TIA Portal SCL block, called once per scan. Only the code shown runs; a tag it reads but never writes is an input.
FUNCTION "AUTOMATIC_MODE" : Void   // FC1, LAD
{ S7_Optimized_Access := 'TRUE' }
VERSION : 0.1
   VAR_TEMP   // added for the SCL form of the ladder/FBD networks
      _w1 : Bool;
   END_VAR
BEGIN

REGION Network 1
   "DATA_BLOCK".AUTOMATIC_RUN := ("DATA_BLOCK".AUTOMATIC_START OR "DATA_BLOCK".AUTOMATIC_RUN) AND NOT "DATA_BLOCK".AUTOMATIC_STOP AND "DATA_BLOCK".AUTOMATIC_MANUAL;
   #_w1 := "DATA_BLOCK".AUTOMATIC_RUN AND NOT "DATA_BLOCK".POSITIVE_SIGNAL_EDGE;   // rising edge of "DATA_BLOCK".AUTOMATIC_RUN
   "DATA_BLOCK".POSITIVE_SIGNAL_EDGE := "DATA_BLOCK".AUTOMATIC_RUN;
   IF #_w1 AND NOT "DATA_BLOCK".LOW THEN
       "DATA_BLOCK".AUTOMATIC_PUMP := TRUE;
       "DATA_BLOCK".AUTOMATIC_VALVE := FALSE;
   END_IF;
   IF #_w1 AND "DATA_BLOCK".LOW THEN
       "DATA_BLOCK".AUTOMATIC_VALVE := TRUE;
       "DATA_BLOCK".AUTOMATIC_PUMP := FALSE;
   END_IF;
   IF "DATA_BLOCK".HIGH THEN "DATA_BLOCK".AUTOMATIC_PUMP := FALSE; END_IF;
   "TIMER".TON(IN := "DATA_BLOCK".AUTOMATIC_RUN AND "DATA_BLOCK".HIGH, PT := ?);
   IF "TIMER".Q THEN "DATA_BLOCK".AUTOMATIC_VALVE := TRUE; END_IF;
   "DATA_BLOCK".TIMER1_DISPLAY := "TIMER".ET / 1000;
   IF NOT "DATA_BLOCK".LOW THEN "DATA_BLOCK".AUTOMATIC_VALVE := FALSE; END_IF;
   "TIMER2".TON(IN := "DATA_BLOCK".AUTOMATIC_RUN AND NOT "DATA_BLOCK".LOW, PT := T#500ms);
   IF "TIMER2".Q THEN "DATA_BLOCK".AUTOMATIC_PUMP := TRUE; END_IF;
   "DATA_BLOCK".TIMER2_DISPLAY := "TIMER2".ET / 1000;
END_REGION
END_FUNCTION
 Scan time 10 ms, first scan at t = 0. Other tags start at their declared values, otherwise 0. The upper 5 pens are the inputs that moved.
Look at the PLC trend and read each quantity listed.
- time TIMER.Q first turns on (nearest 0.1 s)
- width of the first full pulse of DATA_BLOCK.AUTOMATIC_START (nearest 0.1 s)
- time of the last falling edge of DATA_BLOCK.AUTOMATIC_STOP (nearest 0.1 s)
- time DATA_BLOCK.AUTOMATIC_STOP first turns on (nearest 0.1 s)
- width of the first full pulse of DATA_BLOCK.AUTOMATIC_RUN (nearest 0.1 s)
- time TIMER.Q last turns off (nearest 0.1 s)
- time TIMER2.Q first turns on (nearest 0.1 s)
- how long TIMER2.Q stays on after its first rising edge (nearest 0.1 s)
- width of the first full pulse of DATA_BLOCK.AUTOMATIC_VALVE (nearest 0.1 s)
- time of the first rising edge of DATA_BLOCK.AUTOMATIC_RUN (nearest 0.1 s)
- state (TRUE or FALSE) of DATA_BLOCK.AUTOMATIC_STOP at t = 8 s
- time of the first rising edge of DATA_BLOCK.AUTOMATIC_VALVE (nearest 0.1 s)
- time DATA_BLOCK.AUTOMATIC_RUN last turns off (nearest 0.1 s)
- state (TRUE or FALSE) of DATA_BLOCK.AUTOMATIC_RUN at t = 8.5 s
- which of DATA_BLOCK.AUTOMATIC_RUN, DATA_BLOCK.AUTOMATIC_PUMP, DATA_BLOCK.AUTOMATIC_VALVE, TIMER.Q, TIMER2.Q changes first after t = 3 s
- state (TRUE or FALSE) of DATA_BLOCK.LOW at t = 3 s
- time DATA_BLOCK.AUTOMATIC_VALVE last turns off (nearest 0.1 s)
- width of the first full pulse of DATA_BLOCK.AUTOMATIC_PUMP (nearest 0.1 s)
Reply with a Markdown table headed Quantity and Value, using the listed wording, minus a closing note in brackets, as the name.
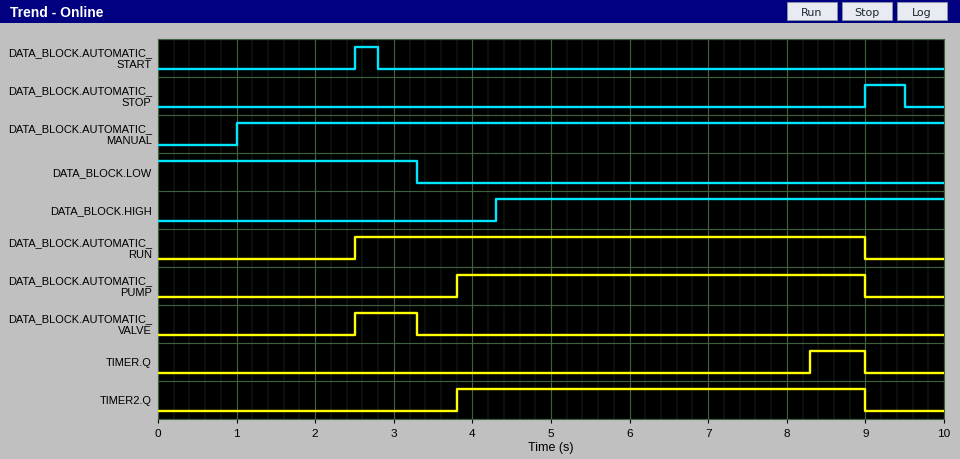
| Quantity | Value |
|---|---|
| time TIMER.Q first turns on | 8.3 s |
| width of the first full pulse of DATA_BLOCK.AUTOMATIC_START | 0.3 s |
| time of the last falling edge of DATA_BLOCK.AUTOMATIC_STOP | 9.5 s |
| time DATA_BLOCK.AUTOMATIC_STOP first turns on | 9.0 s |
| width of the first full pulse of DATA_BLOCK.AUTOMATIC_RUN | 6.5 s |
| time TIMER.Q last turns off | 9.0 s |
| time TIMER2.Q first turns on | 3.8 s |
| how long TIMER2.Q stays on after its first rising edge | 5.2 s |
| width of the first full pulse of DATA_BLOCK.AUTOMATIC_VALVE | 0.8 s |
| time of the first rising edge of DATA_BLOCK.AUTOMATIC_RUN | 2.5 s |
| state (TRUE or FALSE) of DATA_BLOCK.AUTOMATIC_STOP at t = 8 s | FALSE |
| time of the first rising edge of DATA_BLOCK.AUTOMATIC_VALVE | 2.5 s |
| time DATA_BLOCK.AUTOMATIC_RUN last turns off | 9.0 s |
| state (TRUE or FALSE) of DATA_BLOCK.AUTOMATIC_RUN at t = 8.5 s | TRUE |
| which of DATA_BLOCK.AUTOMATIC_RUN, DATA_BLOCK.AUTOMATIC_PUMP, DATA_BLOCK.AUTOMATIC_VALVE, TIMER.Q, TIMER2.Q changes first after t = 3 s | DATA_BLOCK.AUTOMATIC_VALVE |
| state (TRUE or FALSE) of DATA_BLOCK.LOW at t = 3 s | TRUE |
| time DATA_BLOCK.AUTOMATIC_VALVE last turns off | 3.3 s |
| width of the first full pulse of DATA_BLOCK.AUTOMATIC_PUMP | 5.2 s |
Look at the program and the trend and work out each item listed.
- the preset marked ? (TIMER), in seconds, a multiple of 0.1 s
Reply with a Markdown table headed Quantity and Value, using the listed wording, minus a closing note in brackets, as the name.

| Quantity | Value |
|---|---|
| the preset marked ? (TIMER), in seconds, a multiple of 0.1 s | 4.0 s |
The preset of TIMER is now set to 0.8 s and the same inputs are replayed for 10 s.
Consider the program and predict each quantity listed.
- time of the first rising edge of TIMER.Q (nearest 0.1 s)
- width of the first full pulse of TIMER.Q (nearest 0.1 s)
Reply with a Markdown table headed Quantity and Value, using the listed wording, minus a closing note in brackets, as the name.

| Quantity | Value |
|---|---|
| time of the first rising edge of TIMER.Q | 5.1 s |
| width of the first full pulse of TIMER.Q | 3.9 s |
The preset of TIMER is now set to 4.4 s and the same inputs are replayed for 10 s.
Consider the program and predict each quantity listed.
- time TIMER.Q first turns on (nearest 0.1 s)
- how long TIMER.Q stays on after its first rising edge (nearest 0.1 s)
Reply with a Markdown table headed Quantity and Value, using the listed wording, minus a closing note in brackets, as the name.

| Quantity | Value |
|---|---|
| time TIMER.Q first turns on | 8.7 s |
| how long TIMER.Q stays on after its first rising edge | 0.3 s |
